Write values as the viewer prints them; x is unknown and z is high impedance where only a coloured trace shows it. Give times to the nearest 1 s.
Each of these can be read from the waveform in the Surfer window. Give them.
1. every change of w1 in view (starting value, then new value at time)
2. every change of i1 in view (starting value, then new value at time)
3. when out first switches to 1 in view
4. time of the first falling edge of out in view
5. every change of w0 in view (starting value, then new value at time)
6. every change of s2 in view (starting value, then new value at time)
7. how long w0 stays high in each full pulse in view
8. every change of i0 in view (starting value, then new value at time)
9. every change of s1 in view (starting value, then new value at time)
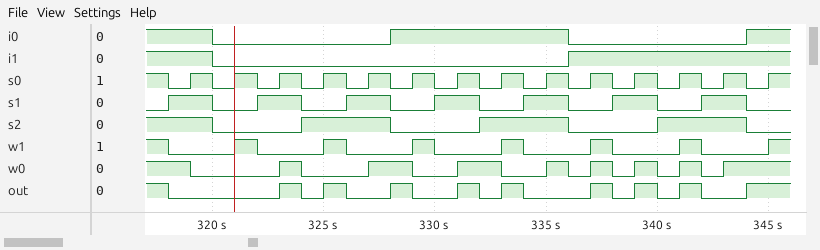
1, 0 at 318 s, 1 at 321 s, 0 at 322 s, 1 at 325 s, 0 at 326 s, 1 at 329 s, 0 at 330 s, 1 at 333 s, 0 at 334 s, 1 at 337 s, 0 at 338 s, 1 at 341 s, 0 at 342 s, 1 at 345 s
1, 0 at 320 s, 1 at 336 s
323 s
318 s
1, 0 at 319 s, 1 at 323 s, 0 at 324 s, 1 at 327 s, 0 at 329 s, 1 at 331 s, 0 at 333 s, 1 at 335 s, 0 at 336 s, 1 at 337 s, 0 at 338 s, 1 at 339 s, 0 at 340 s, 1 at 341 s, 0 at 342 s, 1 at 343 s
1, 0 at 320 s, 1 at 324 s, 0 at 328 s, 1 at 332 s, 0 at 336 s, 1 at 340 s, 0 at 344 s
1 s, 2 s, 2 s, 1 s, 1 s, 1 s, 1 s
1, 0 at 320 s, 1 at 328 s, 0 at 336 s, 1 at 344 s
0, 1 at 318 s, 0 at 320 s, 1 at 322 s, 0 at 324 s, 1 at 326 s, 0 at 328 s, 1 at 330 s, 0 at 332 s, 1 at 334 s, 0 at 336 s, 1 at 338 s, 0 at 340 s, 1 at 342 s, 0 at 344 s
